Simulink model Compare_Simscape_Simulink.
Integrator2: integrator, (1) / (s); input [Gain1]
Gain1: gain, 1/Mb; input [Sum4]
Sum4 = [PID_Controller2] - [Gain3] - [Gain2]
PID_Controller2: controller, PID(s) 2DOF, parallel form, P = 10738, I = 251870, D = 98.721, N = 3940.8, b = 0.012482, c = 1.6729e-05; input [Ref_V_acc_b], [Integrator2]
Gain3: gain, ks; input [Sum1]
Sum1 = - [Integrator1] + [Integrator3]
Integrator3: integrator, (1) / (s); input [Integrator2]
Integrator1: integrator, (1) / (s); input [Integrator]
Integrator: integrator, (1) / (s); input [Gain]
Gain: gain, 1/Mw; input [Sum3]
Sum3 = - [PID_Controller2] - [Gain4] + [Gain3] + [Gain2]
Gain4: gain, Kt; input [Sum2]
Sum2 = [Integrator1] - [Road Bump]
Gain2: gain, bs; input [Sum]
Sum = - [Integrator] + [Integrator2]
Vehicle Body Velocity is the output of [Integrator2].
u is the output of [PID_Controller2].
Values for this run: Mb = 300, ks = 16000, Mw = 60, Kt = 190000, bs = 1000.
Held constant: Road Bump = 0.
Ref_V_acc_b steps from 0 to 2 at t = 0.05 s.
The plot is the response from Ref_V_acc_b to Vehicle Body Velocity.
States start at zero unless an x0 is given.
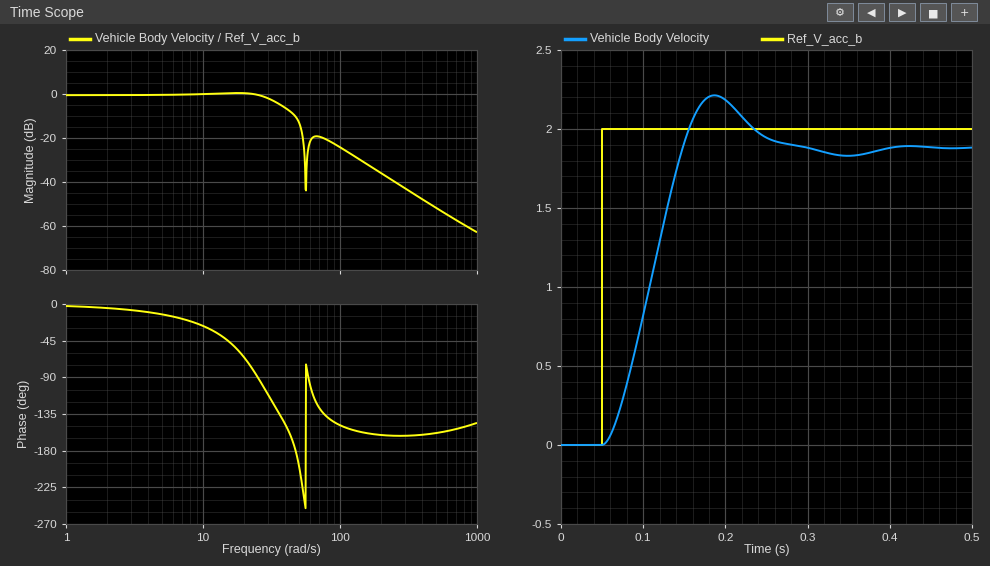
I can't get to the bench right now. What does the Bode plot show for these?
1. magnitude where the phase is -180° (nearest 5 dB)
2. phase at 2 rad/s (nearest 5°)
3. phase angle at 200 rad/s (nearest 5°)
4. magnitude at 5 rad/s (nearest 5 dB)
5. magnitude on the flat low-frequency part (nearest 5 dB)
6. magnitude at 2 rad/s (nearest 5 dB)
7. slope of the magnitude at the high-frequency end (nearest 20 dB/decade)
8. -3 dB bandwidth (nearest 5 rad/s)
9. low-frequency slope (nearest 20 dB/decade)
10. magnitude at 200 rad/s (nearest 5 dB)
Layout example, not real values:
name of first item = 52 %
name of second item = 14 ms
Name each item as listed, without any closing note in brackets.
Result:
magnitude where the phase is -180° = -10 dB
phase at 2 rad/s = -5°
phase angle at 200 rad/s = -160°
magnitude at 5 rad/s = 0 dB
magnitude on the flat low-frequency part = 0 dB
magnitude at 2 rad/s = 0 dB
slope of the magnitude at the high-frequency end = -40 dB/decade
-3 dB bandwidth = 35 rad/s
low-frequency slope = 0 dB/decade
magnitude at 200 rad/s = -35 dB
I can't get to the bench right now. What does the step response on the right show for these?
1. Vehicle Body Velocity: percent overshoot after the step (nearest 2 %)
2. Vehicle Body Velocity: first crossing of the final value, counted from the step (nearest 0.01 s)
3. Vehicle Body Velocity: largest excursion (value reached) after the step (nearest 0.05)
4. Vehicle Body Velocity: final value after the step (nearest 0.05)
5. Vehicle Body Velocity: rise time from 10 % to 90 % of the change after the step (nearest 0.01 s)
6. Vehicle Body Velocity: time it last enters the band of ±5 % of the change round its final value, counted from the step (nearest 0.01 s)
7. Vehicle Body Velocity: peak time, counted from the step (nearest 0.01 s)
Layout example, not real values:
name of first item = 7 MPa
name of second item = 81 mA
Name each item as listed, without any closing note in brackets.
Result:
Vehicle Body Velocity: percent overshoot after the step = 18 %
Vehicle Body Velocity: first crossing of the final value, counted from the step = 0.10 s
Vehicle Body Velocity: largest excursion (value reached) after the step = 2.20
Vehicle Body Velocity: final value after the step = 1.90
Vehicle Body Velocity: rise time from 10 % to 90 % of the change after the step = 0.07 s
Vehicle Body Velocity: time it last enters the band of ±5 % of the change round its final value, counted from the step = 0.19 s
Vehicle Body Velocity: peak time, counted from the step = 0.14 s
